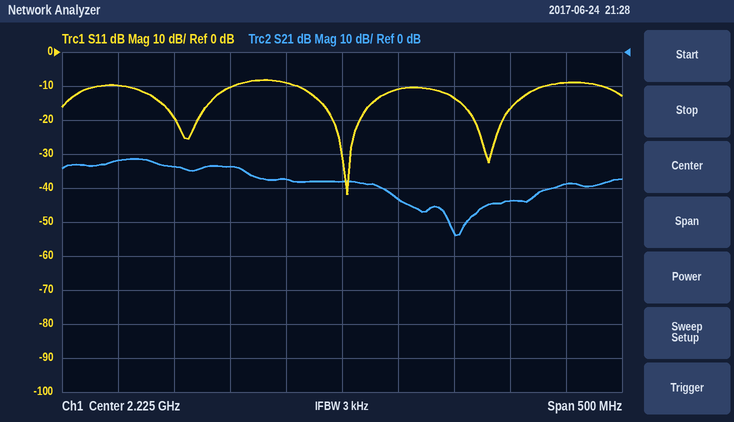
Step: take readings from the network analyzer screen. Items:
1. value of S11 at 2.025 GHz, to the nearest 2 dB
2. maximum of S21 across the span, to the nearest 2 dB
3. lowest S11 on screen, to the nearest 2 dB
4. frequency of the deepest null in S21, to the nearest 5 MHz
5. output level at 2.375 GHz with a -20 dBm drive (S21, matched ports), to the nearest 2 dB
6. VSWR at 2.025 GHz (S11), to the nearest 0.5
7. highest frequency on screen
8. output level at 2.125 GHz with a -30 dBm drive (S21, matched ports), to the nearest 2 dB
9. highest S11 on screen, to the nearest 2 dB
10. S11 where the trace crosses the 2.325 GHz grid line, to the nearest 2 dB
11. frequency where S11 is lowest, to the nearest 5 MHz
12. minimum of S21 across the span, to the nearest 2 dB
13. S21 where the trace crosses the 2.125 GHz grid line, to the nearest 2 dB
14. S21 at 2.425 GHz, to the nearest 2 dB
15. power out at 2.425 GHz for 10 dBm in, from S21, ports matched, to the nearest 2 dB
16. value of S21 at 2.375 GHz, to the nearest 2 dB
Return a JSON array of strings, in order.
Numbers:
["-10 dB", "-32 dB", "-42 dB", "2.325 GHz", "-64 dBm", "2.0", "2.475 GHz", "-64 dBm", "-8 dB", "-14 dB", "2.230 GHz", "-54 dB", "-34 dB", "-38 dB", "-28 dBm", "-44 dB"]
